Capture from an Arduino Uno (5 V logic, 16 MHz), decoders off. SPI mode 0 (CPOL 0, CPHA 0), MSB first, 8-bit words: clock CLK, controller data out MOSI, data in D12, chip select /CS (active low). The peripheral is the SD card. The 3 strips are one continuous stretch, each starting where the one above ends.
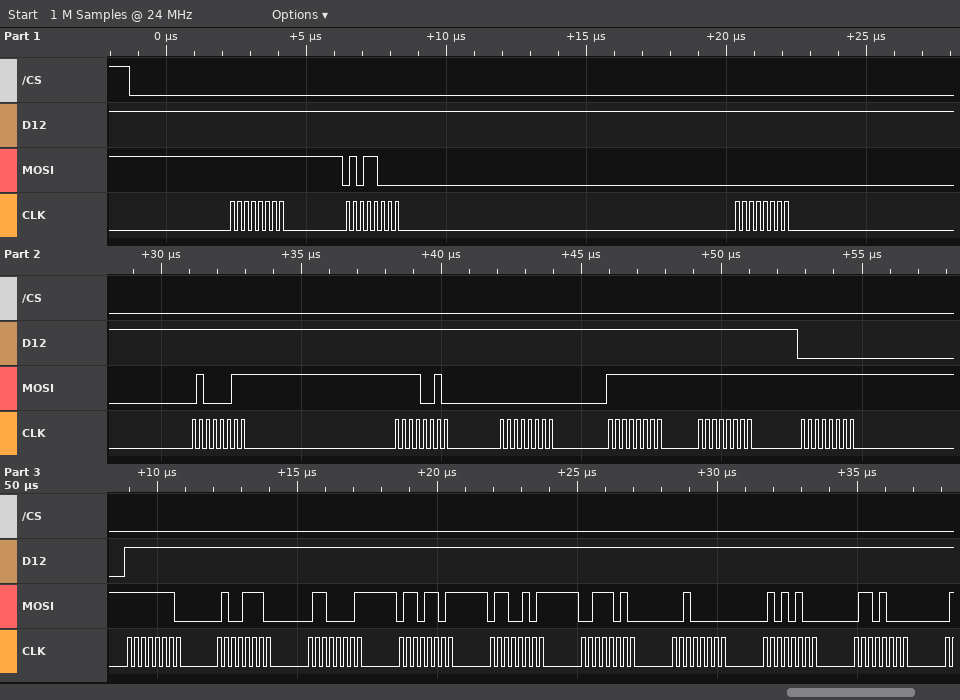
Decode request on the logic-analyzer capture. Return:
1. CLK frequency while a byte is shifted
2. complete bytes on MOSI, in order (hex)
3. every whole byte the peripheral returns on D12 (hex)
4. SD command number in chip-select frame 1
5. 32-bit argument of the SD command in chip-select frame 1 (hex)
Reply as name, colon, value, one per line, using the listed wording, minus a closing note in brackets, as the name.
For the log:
CLK frequency while a byte is shifted: 4 MHz
complete bytes on MOSI, in order: FF 58 00 43 F2 00 FF FF FF FE 4E 61 6D 65 3A 20 54 68
every whole byte the peripheral returns on D12: FF FF FF FF FF FF FF FF 00 FF FF FF FF FF FF FF FF FF
SD command number in chip-select frame 1: CMD24
32-bit argument of the SD command in chip-select frame 1: 0x0043F200
